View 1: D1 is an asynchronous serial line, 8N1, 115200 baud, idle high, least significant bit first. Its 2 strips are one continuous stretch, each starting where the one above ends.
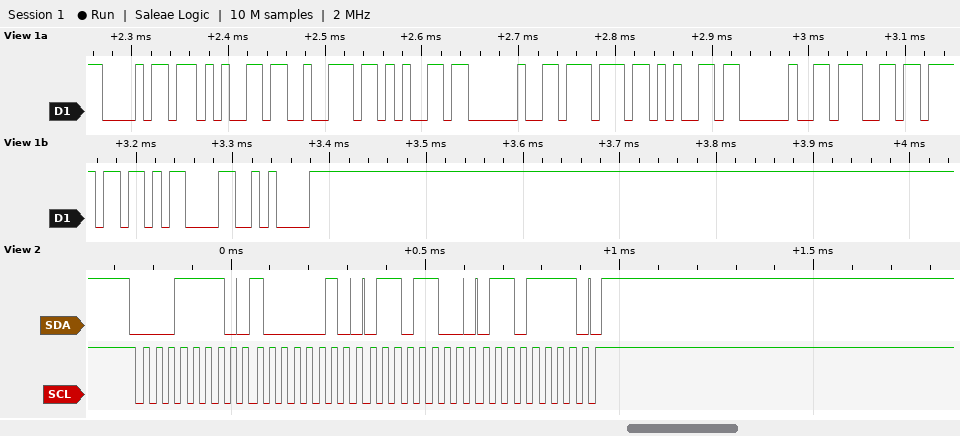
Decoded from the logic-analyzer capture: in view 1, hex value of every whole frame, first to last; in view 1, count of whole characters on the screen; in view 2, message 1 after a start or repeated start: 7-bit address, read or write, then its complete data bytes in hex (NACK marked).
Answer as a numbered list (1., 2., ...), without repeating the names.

1. 68 65 72 65 20 77 65 20 67 6F 0D 0A
2. 12
3. 0x0F write: 82 6C 6F
